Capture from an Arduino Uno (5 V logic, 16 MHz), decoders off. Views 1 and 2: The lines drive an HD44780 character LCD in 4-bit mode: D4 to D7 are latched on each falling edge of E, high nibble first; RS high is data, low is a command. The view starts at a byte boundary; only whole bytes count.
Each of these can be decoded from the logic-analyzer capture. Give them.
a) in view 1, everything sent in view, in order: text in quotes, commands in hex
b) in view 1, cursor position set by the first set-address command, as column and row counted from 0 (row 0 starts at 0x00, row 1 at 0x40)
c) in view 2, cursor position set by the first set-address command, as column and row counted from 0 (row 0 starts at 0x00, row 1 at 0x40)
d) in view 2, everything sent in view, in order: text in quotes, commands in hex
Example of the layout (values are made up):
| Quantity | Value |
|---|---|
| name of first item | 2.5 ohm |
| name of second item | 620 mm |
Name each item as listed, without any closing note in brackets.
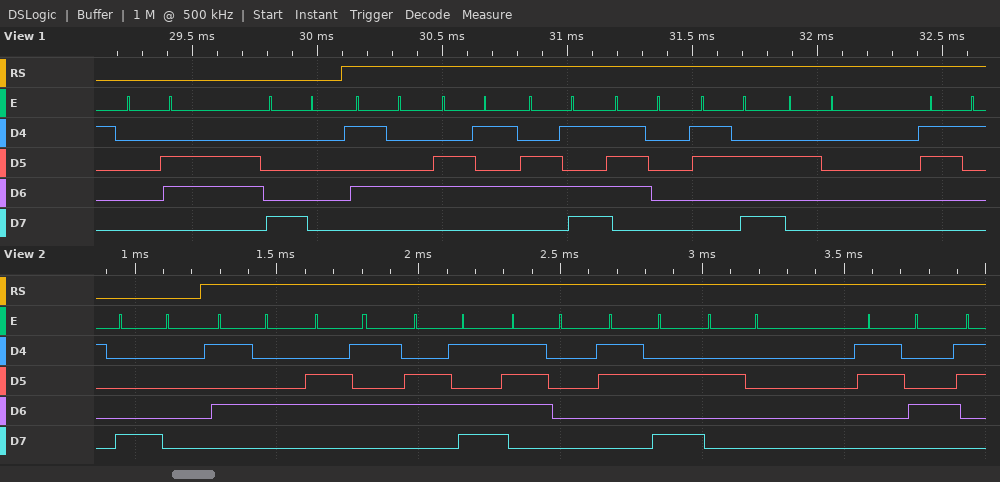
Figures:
| Quantity | Value |
|---|---|
| in view 1, everything sent in view, in order: text in quotes, commands in hex | 0x06 0x80 "Temp: 1" |
| in view 1, cursor position set by the first set-address command, as column and row counted from 0 | column 0, row 0 |
| in view 2, cursor position set by the first set-address command, as column and row counted from 0 | column 0, row 0 |
| in view 2, everything sent in view, in order: text in quotes, commands in hex | 0x80 "Temp: 4" |
